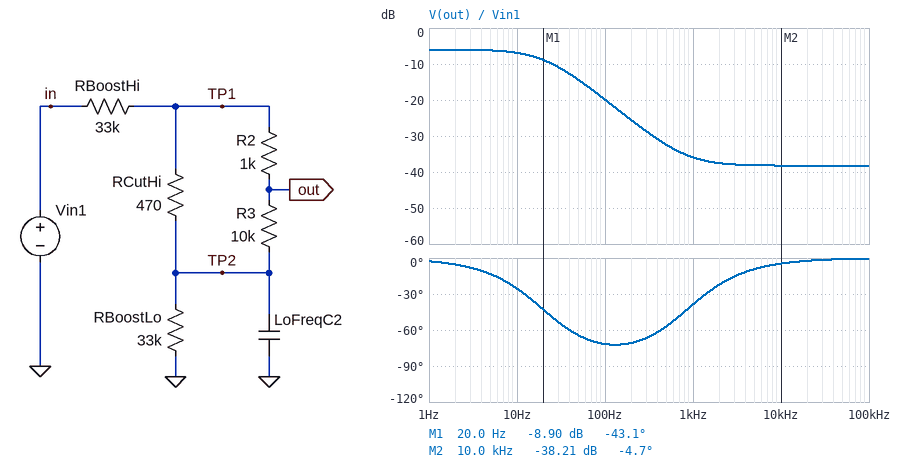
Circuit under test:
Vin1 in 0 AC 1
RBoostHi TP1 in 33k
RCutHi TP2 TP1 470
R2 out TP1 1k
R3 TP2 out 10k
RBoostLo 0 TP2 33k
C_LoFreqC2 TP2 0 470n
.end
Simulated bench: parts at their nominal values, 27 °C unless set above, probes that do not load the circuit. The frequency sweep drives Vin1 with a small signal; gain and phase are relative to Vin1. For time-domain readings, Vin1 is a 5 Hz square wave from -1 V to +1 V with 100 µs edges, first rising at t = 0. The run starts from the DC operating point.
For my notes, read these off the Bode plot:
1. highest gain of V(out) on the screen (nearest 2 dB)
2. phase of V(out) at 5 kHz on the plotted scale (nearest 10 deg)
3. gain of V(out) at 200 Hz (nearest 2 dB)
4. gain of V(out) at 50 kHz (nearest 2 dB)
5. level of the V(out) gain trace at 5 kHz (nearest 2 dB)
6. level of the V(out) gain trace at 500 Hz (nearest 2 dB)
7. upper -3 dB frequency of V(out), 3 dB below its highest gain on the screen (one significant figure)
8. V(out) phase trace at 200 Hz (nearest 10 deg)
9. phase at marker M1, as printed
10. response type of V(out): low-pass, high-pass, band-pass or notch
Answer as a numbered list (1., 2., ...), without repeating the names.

1. -6 dB
2. -10 deg
3. -26 dB
4. -38 dB
5. -38 dB
6. -32 dB
7. 20 Hz
8. -70 deg
9. -43.1 deg
10. low-pass
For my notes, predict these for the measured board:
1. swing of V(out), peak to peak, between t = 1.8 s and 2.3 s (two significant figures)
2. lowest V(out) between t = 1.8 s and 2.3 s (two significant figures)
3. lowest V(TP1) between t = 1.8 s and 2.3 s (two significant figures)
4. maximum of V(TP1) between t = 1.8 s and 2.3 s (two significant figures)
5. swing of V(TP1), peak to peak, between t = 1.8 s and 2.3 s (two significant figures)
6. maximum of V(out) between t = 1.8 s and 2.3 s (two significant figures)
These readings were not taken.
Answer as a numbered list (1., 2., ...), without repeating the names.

1. 1.0 V
2. -500 mV
3. -500 mV
4. 500 mV
5. 1.0 V
6. 500 mV
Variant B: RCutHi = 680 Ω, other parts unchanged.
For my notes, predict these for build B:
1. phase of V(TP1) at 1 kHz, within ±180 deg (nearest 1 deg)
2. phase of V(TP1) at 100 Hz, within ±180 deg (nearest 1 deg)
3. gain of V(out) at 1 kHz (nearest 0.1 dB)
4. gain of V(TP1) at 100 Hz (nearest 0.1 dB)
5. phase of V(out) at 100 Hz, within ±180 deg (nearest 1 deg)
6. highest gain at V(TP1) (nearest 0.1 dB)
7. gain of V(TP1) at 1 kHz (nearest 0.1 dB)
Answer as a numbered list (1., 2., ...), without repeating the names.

1. -27 deg
2. -68 deg
3. -33.9 dB
4. -19.8 dB
5. -69 deg
6. -5.9 dB
7. -33.3 dB
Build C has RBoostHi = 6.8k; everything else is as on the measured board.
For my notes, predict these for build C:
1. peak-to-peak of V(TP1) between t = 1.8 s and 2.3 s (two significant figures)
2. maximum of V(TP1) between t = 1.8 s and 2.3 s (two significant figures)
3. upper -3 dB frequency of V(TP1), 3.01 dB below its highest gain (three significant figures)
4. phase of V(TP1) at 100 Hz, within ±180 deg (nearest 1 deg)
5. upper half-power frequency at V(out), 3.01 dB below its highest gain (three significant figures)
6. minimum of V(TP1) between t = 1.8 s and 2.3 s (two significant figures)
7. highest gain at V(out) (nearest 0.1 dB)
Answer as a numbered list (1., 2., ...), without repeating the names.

1. 1.7 V
2. 830 mV
3. 57.3 Hz
4. -53 deg
5. 57.2 Hz
6. -830 mV
7. -1.6 dB
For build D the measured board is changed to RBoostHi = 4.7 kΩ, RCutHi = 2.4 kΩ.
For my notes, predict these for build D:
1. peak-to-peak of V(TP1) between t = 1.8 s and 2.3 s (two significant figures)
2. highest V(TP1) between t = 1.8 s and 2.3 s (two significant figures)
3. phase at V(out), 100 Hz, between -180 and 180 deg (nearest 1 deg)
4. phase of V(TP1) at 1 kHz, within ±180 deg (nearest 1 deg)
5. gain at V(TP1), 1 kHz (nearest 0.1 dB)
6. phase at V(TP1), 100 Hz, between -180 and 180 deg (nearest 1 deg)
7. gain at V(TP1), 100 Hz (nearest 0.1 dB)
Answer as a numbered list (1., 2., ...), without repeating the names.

1. 1.8 V
2. 880 mV
3. -32 deg
4. -7 deg
5. -10.5 dB
6. -30 deg
7. -5.6 dB
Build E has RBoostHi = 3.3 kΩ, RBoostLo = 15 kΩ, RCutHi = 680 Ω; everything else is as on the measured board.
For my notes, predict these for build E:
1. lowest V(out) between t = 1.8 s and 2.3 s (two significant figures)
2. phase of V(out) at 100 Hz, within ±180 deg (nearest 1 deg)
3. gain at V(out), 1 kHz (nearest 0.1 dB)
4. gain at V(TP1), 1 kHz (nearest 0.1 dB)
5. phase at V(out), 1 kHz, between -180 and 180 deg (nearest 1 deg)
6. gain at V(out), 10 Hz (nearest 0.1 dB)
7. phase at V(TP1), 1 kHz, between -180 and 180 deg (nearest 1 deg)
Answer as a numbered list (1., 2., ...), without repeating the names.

1. -820 mV
2. -33 deg
3. -15.3 dB
4. -14.7 dB
5. -25 deg
6. -1.7 dB
7. -23 deg
